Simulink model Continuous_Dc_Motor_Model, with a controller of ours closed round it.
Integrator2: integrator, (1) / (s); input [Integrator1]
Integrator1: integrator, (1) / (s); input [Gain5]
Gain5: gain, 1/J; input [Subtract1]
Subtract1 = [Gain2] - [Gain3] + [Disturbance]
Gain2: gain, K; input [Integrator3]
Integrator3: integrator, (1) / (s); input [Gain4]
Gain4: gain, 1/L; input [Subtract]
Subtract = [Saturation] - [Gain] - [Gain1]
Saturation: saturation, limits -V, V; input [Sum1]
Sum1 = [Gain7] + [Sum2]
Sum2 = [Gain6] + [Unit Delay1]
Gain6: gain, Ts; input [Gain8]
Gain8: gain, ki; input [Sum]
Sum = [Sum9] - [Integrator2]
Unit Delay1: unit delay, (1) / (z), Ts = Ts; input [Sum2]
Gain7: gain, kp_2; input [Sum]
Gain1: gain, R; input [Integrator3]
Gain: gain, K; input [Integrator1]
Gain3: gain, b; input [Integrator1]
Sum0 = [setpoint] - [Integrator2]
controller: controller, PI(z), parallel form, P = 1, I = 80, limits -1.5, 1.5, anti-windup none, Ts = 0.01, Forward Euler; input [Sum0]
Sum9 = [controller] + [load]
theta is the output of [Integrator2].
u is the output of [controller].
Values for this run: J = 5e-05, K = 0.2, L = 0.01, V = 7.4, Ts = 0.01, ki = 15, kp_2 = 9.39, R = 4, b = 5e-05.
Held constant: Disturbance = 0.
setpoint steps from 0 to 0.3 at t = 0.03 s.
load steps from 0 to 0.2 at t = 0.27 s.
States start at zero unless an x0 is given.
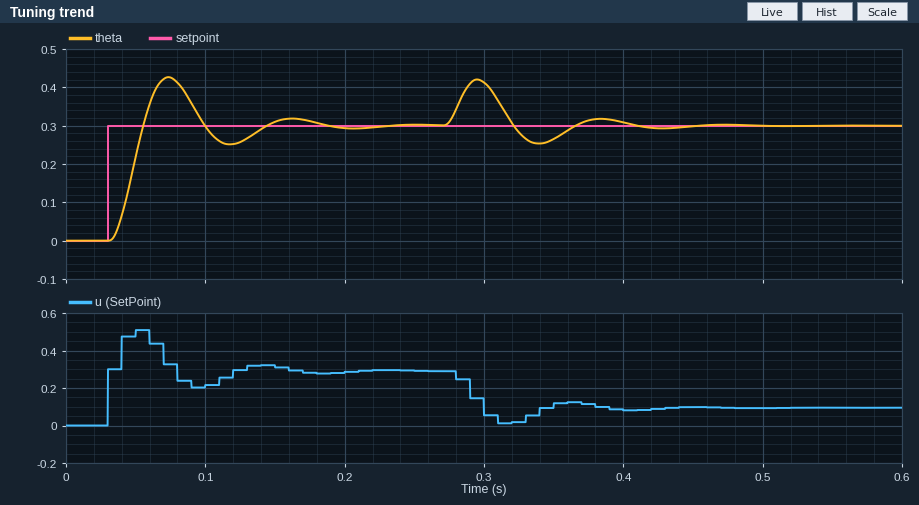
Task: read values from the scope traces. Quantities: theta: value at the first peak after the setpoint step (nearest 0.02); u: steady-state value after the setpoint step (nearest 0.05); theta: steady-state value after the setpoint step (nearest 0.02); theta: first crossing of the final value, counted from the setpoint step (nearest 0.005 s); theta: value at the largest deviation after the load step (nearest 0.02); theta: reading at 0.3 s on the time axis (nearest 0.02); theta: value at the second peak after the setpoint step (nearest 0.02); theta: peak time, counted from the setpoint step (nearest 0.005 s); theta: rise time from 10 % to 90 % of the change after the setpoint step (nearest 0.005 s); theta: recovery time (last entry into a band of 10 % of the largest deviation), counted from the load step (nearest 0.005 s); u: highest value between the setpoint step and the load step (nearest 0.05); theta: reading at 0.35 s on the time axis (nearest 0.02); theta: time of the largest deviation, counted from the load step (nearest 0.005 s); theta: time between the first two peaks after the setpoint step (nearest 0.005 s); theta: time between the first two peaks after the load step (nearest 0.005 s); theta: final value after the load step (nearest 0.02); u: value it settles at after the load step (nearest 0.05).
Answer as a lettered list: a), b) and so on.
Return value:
a) 0.42
b) 0.30
c) 0.30
d) 0.025 s
e) 0.42
f) 0.42
g) 0.32
h) 0.045 s
i) 0.015 s
j) 0.125 s
k) 0.50
l) 0.26
m) 0.025 s
n) 0.090 s
o) 0.090 s
p) 0.30
q) 0.10
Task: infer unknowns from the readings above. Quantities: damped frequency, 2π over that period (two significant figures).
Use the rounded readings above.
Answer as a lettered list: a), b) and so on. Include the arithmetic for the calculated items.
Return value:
a) 2π / 0.09 = 70 rad/s
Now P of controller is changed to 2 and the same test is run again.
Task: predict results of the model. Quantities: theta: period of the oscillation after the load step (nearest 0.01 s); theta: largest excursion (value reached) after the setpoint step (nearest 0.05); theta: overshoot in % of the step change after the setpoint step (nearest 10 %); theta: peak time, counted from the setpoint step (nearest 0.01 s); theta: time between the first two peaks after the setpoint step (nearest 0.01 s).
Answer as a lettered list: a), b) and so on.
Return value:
a) 0.05 s
b) 0.40
c) 40 %
d) 0.03 s
e) 0.05 s
